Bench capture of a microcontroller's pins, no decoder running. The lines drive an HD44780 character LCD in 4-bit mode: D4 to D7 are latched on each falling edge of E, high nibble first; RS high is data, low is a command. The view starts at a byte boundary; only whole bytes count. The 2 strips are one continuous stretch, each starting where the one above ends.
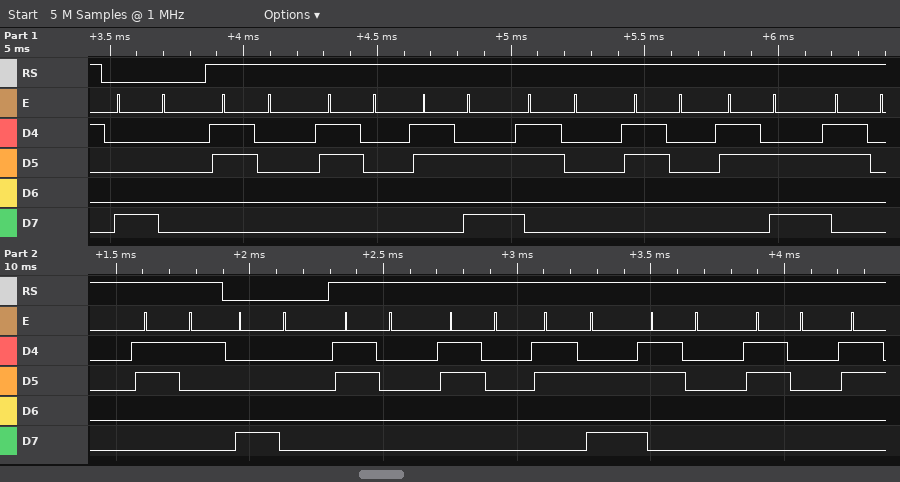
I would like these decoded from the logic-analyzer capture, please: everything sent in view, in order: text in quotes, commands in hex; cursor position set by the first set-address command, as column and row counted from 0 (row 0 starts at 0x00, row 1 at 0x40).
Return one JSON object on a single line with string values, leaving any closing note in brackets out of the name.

{"everything sent in view, in order: text in quotes, commands in hex": "0x80 \"00:00:01\" 0x80 \"00:00\"", "cursor position set by the first set-address command, as column and row counted from 0": "column 0, row 0"}
